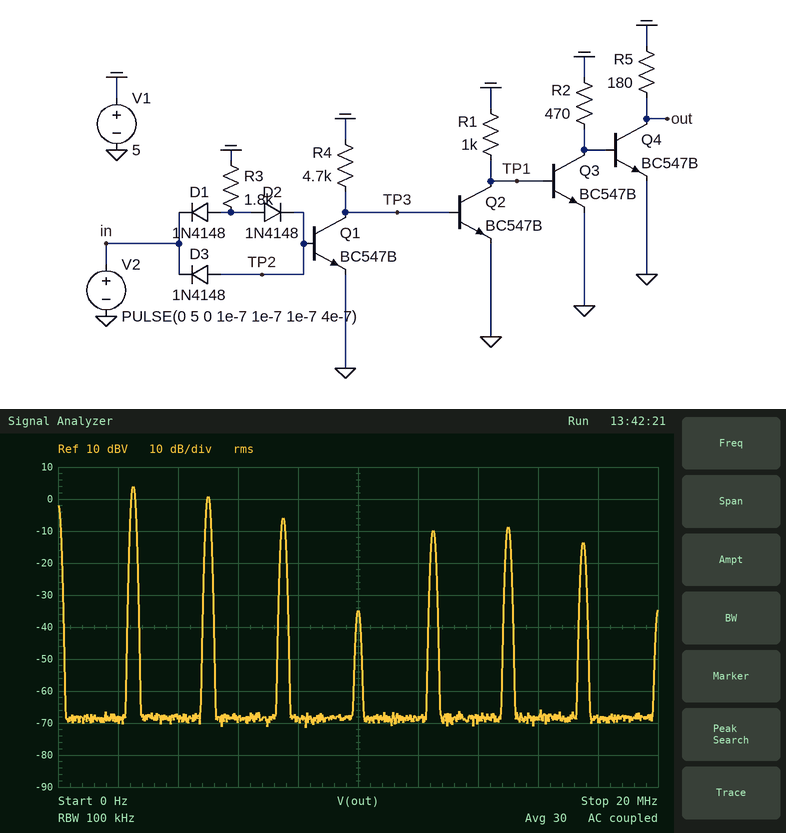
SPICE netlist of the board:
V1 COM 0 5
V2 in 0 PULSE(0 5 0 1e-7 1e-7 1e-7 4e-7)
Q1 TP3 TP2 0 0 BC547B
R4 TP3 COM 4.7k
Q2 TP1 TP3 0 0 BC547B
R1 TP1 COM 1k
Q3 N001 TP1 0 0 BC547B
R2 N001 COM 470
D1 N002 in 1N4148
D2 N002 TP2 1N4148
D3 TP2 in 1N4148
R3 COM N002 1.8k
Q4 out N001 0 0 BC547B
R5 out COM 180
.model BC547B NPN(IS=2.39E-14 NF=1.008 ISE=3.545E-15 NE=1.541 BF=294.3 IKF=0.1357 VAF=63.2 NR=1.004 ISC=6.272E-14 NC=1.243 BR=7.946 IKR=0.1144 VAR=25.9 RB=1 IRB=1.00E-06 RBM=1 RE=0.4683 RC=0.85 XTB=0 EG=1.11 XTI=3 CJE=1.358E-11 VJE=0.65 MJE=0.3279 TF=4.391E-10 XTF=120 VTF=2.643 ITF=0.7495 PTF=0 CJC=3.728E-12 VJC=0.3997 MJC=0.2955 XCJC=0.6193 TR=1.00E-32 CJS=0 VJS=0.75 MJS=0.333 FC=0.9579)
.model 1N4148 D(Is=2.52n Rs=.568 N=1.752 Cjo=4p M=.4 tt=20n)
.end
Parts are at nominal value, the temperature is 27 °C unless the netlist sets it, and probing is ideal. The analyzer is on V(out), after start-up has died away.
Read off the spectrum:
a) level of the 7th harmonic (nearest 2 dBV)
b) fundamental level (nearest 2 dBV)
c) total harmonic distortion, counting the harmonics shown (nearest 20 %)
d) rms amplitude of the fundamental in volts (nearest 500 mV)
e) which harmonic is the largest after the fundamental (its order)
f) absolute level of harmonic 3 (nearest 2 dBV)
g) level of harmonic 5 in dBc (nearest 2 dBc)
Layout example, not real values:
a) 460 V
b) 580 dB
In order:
a) -14 dBV
b) 4 dBV
c) 80 %
d) 1.5 V
e) 2
f) -6 dBV
g) -14 dBc
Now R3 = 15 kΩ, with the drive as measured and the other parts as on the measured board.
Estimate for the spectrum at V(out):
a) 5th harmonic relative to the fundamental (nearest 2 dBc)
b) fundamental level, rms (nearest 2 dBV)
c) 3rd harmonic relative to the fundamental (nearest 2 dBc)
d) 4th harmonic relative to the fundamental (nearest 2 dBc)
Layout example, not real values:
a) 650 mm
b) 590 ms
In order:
a) -12 dBc
b) 4 dBV
c) -12 dBc
d) -22 dBc
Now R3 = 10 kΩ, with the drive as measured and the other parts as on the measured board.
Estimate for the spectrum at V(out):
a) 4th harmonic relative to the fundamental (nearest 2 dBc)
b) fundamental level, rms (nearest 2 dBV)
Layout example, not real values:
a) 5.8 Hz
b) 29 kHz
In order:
a) -30 dBc
b) 4 dBV
